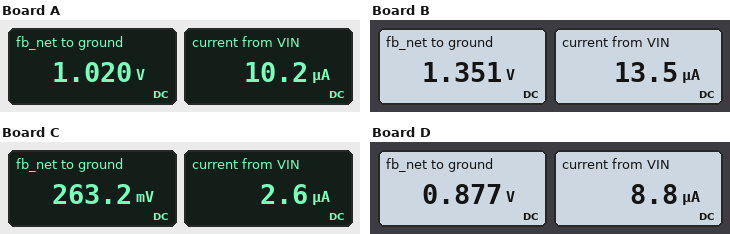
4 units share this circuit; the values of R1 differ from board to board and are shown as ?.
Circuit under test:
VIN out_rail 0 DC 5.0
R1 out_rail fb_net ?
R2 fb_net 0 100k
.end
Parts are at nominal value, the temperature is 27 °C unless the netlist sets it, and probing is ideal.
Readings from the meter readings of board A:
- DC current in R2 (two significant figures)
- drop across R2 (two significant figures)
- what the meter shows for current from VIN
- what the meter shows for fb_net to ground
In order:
10 µA
1.0 V
10.2 µA
1.020 V
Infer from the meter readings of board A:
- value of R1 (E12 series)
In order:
390 kΩ
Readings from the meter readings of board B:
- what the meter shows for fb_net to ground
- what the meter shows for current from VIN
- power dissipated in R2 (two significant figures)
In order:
1.351 V
13.5 µA
18 µW
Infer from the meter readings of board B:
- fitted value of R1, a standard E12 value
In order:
270 kΩ
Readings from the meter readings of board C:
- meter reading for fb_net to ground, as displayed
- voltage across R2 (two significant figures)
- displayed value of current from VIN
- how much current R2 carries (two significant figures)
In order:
263.2 mV
260 mV
2.6 µA
2.6 µA
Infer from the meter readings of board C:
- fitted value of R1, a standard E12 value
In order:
1.8 MΩ
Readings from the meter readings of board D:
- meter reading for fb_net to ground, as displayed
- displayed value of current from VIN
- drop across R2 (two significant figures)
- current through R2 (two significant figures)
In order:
0.877 V
8.8 µA
880 mV
8.8 µA
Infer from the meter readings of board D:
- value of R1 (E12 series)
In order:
470 kΩ
